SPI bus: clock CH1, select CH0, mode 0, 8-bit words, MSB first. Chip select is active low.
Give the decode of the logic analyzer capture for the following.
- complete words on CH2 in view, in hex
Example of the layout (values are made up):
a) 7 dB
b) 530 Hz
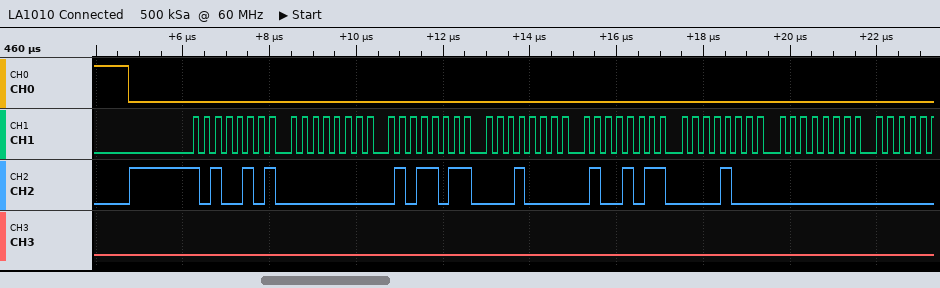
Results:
a) A5, 00, 5B, 10, 4B, 08, 00
